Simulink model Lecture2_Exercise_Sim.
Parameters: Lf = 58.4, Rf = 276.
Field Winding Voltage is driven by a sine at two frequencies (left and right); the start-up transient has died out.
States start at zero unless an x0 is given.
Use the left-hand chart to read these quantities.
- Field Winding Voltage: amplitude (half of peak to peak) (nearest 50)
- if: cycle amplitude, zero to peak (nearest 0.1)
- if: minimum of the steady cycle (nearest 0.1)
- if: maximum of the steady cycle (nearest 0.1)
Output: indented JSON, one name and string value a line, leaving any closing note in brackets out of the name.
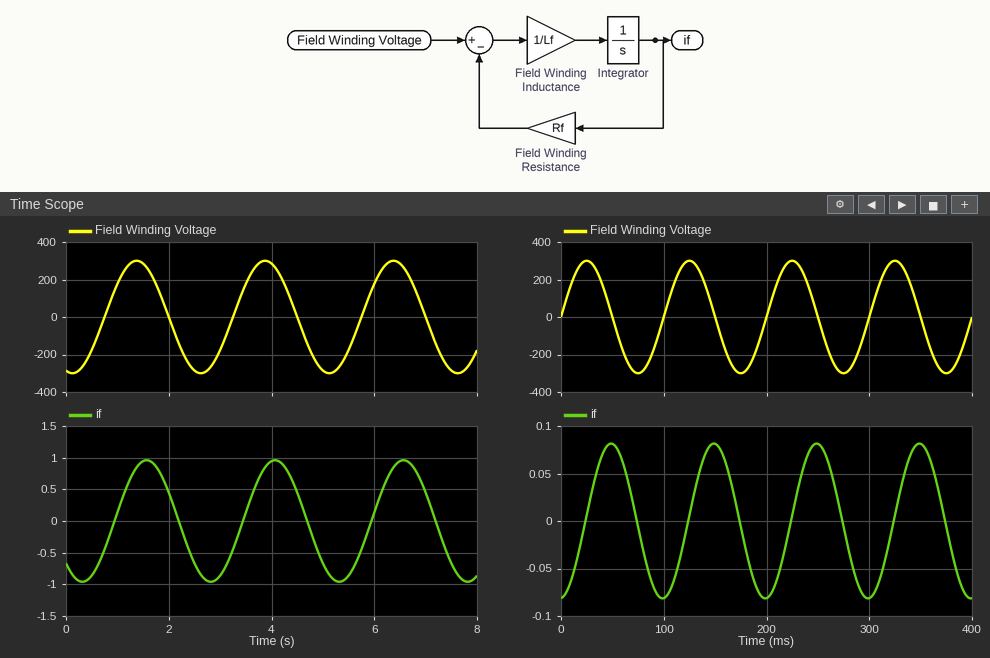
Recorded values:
{
  "Field Winding Voltage: amplitude (half of peak to peak)": "300",
  "if: cycle amplitude, zero to peak": "1.0",
  "if: minimum of the steady cycle": "-1.0",
  "if: maximum of the steady cycle": "1.0"
}
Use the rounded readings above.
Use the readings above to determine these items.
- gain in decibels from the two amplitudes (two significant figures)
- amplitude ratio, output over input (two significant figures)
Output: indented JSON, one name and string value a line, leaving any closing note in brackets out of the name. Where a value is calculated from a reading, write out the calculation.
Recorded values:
{
  "gain in decibels from the two amplitudes": "20 log10(1 / 300) = -50 dB",
  "amplitude ratio, output over input": "1 / 300 = 0.0033"
}
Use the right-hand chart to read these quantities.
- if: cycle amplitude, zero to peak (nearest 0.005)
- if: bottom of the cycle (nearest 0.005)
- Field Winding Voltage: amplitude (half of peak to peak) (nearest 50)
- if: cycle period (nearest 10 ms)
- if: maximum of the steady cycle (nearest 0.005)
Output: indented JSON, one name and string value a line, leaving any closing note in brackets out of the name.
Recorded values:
{
  "if: cycle amplitude, zero to peak": "0.080",
  "if: bottom of the cycle": "-0.080",
  "Field Winding Voltage: amplitude (half of peak to peak)": "300",
  "if: cycle period": "100 ms",
  "if: maximum of the steady cycle": "0.080"
}
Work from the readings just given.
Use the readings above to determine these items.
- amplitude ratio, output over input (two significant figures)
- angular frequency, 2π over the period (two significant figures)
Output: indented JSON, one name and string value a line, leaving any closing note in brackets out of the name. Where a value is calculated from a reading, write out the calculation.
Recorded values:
{
  "amplitude ratio, output over input": "0.08 / 300 = 0.00027",
  "angular frequency, 2π over the period": "2π / 100 = 0.063 rad/ms"
}
